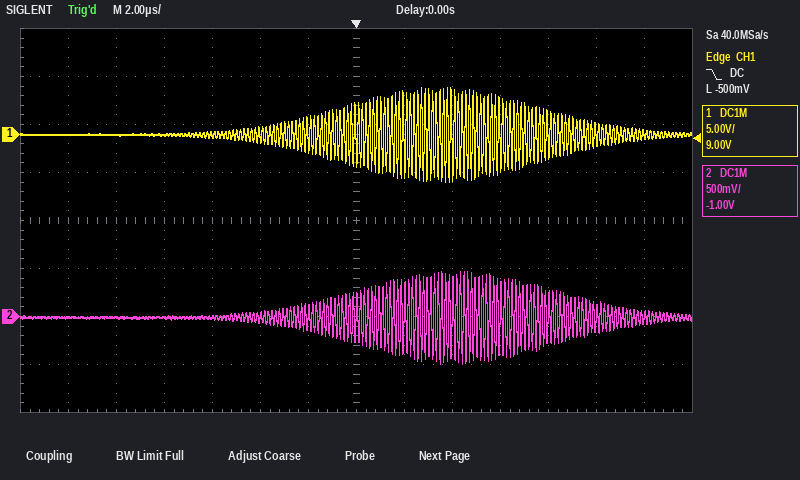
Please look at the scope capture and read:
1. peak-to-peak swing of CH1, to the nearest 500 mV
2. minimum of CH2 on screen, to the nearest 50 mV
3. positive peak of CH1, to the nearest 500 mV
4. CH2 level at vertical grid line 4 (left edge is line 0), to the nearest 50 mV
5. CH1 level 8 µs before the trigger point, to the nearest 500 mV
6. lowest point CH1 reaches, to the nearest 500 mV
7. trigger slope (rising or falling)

10.0 V
-500 mV
5.0 V
0 mV
0.0 V
-5.0 V
falling
